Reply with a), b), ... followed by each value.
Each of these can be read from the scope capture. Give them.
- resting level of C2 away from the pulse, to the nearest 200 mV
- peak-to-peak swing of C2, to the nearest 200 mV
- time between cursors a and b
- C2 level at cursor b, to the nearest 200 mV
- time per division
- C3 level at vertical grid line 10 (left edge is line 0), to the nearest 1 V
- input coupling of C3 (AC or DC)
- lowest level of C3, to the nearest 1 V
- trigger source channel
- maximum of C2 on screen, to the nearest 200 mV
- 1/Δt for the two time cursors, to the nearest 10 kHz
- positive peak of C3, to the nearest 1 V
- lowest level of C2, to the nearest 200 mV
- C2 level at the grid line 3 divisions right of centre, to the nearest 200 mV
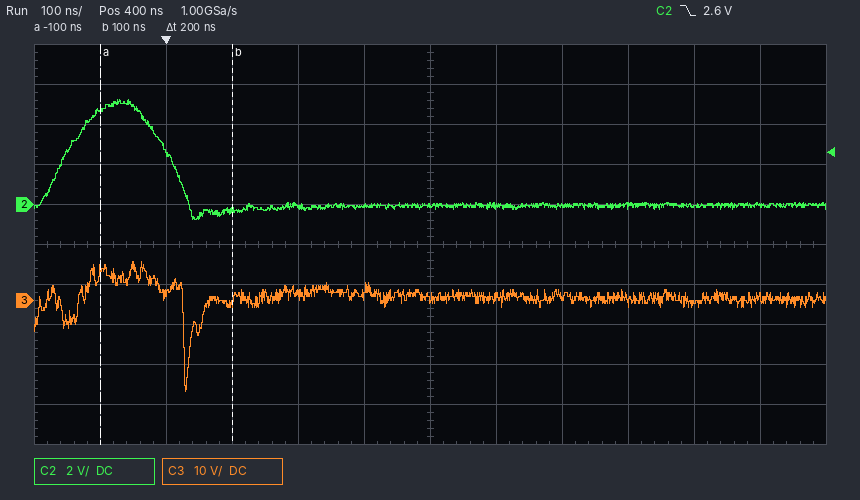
a) 0.0 V
b) 6.0 V
c) 200 ns
d) -400 mV
e) 100 ns
f) -1 V
g) DC
h) -23 V
i) C2
j) 5.2 V
k) 5.00 MHz
l) 10 V
m) -800 mV
n) 0.0 V
